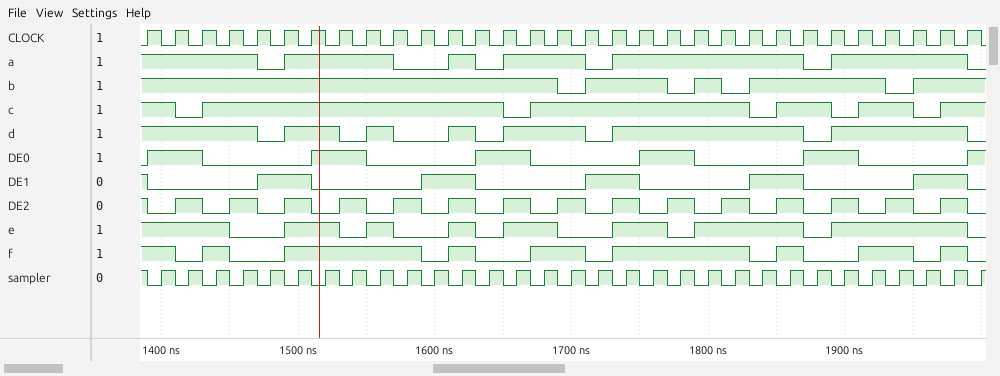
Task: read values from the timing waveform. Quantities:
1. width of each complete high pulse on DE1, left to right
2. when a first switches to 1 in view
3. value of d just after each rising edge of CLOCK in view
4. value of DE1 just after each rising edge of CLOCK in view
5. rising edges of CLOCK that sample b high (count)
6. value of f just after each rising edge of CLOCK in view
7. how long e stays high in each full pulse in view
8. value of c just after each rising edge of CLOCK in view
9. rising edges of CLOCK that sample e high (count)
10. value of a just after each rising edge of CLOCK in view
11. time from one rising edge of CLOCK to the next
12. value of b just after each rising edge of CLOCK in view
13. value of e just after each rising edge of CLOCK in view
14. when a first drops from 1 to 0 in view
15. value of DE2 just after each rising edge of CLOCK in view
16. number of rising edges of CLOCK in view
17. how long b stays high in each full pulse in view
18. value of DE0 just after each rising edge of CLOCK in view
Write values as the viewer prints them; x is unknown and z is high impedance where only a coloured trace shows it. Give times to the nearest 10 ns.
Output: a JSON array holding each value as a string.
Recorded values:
["40 ns, 40 ns, 40 ns, 40 ns, 40 ns", "1490 ns", "1 1 1 1 0 1 1 0 1 0 0 1 0 1 1 1 0 1 1 1 1 1 1 1 0 1 1 1 1 1 0", "0 0 0 0 1 1 0 0 0 0 1 1 0 0 0 0 1 1 0 0 0 0 1 1 0 0 0 0 1 1 0", "27", "1 0 1 0 0 1 1 1 1 1 0 1 0 0 1 1 0 1 1 1 1 1 0 1 0 0 1 1 0 1 0", "40 ns, 20 ns, 20 ns, 40 ns, 40 ns, 80 ns, 100 ns", "1 0 1 1 1 1 1 1 1 1 1 1 1 0 1 1 1 1 1 1 1 1 0 1 1 0 1 1 0 1 1", "21", "1 1 1 1 0 1 1 1 1 0 0 1 0 1 1 1 0 1 1 1 1 1 1 1 0 1 1 1 1 1 0", "20 ns", "1 1 1 1 1 1 1 1 1 1 1 1 1 1 1 0 1 1 1 0 1 0 1 1 1 1 1 0 1 1 1", "1 1 1 0 0 1 1 0 1 0 0 1 0 1 1 0 0 1 1 0 1 1 1 1 0 1 1 1 1 1 0", "1470 ns", "0 1 0 1 0 1 0 1 0 1 0 1 0 1 0 1 0 1 0 1 0 1 0 1 0 1 0 1 0 1 0", "31", "60 ns, 20 ns, 100 ns", "1 1 0 0 0 0 1 1 0 0 0 0 1 1 0 0 0 0 1 1 0 0 0 0 1 1 0 0 0 0 1"]
